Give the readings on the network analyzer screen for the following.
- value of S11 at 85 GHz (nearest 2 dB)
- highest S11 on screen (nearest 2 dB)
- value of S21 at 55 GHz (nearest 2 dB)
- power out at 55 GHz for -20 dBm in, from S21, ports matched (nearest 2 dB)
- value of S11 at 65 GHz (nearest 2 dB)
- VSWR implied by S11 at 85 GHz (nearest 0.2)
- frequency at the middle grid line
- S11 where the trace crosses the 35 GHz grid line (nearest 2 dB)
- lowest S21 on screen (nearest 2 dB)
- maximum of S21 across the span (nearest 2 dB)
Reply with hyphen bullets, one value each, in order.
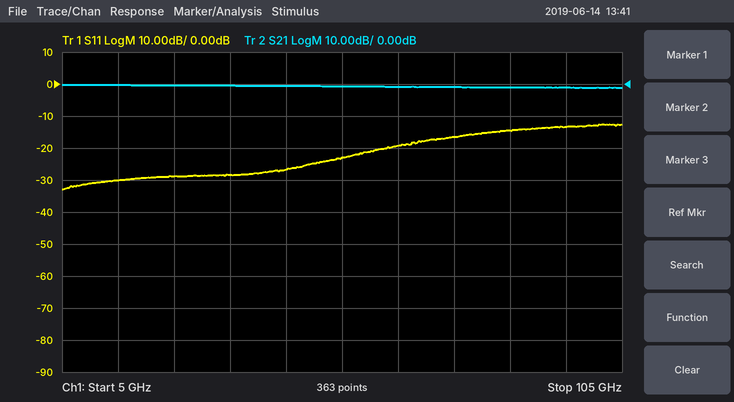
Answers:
- -14 dB
- -12 dB
- 0 dB
- -20 dBm
- -20 dB
- 1.4
- 55 GHz
- -28 dB
- -2 dB
- 0 dB
